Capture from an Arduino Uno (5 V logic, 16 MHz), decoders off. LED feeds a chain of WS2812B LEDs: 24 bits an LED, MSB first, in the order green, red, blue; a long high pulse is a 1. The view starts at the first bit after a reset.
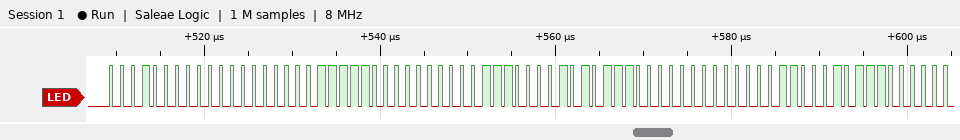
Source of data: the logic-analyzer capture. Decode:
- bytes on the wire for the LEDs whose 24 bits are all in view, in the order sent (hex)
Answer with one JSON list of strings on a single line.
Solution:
["10 00 1F 00 38 57 00 06 2E"]
